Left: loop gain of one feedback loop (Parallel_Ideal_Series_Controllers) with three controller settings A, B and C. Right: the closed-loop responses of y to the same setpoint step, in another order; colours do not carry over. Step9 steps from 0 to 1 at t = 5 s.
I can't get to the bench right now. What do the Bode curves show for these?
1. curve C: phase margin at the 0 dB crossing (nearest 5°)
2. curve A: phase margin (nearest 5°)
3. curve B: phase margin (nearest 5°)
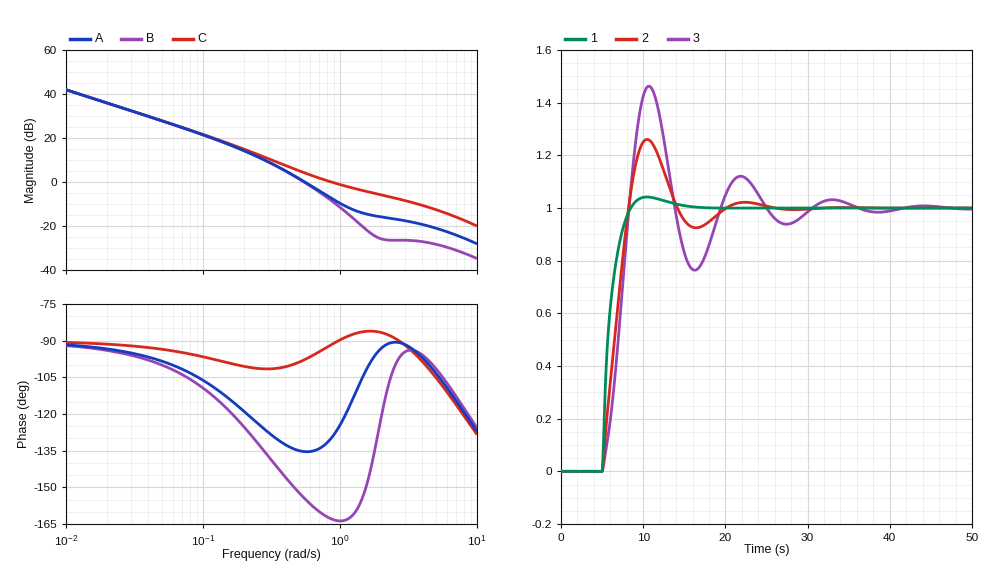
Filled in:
90°
45°
25°
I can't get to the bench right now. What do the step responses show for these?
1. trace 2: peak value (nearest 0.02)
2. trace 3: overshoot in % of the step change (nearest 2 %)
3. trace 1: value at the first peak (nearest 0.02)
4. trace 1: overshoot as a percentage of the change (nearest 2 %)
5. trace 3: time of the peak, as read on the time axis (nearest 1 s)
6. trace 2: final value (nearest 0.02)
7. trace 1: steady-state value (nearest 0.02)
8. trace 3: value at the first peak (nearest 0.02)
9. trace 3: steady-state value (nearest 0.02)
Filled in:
1.26
46 %
1.04
4 %
11 s
1.00
1.00
1.46
1.00
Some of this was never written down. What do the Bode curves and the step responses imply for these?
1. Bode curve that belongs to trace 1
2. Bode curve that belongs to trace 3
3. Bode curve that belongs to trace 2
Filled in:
C
B
A
